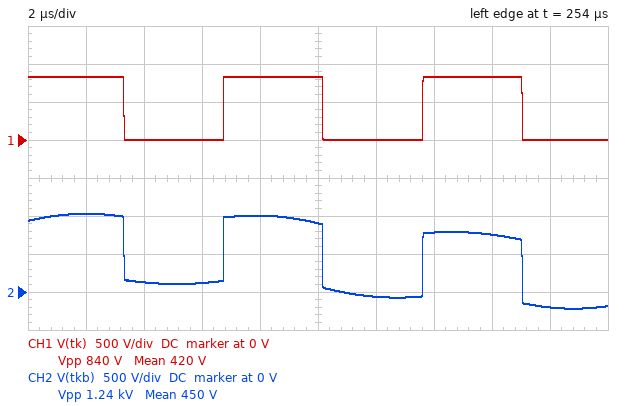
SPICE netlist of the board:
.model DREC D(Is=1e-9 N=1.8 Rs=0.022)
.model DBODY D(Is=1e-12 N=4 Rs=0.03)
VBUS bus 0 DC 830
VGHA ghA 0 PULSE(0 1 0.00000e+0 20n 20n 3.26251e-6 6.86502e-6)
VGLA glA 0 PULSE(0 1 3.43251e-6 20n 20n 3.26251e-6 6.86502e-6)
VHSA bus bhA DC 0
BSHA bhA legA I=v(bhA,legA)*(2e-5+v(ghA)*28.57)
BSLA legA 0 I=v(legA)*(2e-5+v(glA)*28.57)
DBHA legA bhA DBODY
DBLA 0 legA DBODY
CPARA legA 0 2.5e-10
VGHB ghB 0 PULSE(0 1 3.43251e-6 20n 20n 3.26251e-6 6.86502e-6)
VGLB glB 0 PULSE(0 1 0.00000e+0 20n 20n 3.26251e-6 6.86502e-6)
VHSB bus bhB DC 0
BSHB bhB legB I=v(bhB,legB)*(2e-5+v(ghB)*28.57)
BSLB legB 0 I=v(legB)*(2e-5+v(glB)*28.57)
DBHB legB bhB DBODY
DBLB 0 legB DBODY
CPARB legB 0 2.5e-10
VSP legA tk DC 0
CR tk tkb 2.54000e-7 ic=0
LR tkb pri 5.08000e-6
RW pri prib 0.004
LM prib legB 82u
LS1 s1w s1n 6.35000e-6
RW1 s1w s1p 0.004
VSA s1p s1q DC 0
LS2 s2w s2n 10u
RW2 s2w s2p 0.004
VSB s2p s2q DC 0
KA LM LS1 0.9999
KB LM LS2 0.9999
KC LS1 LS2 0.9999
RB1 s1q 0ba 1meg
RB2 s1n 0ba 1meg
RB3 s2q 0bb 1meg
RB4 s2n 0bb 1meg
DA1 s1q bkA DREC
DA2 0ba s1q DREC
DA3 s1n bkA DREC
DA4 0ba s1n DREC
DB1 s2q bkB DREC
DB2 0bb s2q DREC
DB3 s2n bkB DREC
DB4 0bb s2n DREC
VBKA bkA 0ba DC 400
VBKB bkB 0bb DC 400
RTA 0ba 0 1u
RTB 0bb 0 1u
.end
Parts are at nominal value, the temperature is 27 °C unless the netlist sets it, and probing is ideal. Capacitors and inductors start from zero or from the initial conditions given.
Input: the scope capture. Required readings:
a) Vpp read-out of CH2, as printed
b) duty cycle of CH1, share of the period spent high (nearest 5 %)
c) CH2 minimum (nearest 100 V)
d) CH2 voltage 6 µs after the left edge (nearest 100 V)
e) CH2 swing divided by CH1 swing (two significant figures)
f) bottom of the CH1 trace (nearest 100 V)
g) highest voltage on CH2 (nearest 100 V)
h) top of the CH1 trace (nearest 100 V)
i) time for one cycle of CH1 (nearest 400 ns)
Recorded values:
1.24 kV
50 %
-200 V
100 V
1.5
0 V
1.0 kV
800 V
6.8 µs
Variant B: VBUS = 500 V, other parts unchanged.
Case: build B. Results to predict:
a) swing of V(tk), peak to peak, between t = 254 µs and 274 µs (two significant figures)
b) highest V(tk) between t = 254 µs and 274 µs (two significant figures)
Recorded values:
510 V
500 V
